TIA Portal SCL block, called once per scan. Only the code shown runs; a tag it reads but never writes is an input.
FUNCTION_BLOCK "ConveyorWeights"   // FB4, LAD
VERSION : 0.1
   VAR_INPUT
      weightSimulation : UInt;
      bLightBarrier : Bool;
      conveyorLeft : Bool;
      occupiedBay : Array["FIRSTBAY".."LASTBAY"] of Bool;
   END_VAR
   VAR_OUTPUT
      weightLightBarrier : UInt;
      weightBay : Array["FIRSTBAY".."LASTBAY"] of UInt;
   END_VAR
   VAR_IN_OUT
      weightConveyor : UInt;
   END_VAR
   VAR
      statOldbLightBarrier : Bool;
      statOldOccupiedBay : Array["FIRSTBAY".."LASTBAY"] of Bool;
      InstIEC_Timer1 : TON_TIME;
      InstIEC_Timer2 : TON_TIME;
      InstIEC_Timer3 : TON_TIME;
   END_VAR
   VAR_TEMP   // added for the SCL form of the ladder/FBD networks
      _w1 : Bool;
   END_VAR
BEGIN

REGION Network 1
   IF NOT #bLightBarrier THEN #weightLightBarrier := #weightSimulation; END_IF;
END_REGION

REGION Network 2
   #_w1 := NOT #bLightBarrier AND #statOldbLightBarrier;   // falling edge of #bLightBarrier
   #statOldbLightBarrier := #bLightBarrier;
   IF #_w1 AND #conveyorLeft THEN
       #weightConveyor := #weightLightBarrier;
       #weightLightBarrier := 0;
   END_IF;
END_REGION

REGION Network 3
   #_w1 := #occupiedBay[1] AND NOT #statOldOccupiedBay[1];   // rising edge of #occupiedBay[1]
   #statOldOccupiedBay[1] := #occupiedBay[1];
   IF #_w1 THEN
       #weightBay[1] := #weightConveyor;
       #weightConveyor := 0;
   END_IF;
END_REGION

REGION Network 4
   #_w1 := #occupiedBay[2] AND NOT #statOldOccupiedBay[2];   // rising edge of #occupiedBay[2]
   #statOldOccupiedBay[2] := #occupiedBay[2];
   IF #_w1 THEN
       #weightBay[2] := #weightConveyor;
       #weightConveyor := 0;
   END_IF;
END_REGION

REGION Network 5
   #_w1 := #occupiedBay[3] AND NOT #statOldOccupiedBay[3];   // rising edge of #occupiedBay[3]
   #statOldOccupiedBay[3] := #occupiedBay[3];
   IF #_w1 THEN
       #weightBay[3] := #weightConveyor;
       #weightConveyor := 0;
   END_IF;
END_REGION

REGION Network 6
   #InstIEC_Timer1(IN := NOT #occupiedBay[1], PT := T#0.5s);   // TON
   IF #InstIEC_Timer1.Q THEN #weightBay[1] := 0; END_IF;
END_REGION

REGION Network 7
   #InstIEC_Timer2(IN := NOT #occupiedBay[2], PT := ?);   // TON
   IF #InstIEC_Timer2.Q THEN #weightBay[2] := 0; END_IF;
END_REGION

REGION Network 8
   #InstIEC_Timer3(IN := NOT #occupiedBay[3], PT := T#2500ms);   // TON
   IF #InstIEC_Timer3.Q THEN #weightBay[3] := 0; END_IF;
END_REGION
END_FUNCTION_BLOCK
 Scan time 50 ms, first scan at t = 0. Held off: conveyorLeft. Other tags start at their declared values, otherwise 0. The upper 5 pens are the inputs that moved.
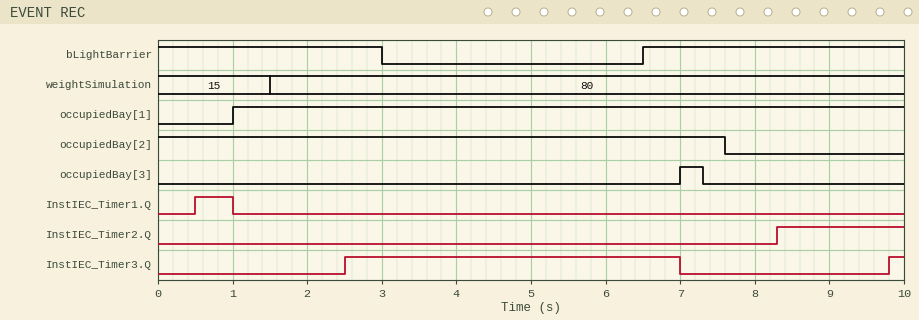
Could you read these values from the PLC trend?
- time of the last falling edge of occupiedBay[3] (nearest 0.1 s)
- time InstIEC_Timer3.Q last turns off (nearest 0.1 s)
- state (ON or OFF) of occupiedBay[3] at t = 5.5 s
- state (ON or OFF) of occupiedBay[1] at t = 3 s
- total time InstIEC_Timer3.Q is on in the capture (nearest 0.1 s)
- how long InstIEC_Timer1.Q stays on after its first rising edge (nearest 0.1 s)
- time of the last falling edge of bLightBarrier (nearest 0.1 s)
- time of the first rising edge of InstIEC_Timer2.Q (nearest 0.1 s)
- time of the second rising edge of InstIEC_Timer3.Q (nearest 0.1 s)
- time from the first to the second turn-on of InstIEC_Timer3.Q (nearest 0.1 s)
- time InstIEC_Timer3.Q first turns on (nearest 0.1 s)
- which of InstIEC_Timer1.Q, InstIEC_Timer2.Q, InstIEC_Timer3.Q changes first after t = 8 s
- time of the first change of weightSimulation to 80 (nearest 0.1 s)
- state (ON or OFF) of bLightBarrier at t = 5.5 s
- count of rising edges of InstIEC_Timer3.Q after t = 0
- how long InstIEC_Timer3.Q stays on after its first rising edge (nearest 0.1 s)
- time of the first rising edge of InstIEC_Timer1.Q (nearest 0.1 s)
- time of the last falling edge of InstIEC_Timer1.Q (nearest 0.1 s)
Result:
7.3 s
7.0 s
OFF
ON
4.7 s
0.5 s
3.0 s
8.3 s
9.8 s
7.3 s
2.5 s
InstIEC_Timer2.Q
1.5 s
OFF
2
4.5 s
0.5 s
1.0 s
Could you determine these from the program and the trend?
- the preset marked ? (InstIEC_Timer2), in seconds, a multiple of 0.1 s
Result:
0.7 s
